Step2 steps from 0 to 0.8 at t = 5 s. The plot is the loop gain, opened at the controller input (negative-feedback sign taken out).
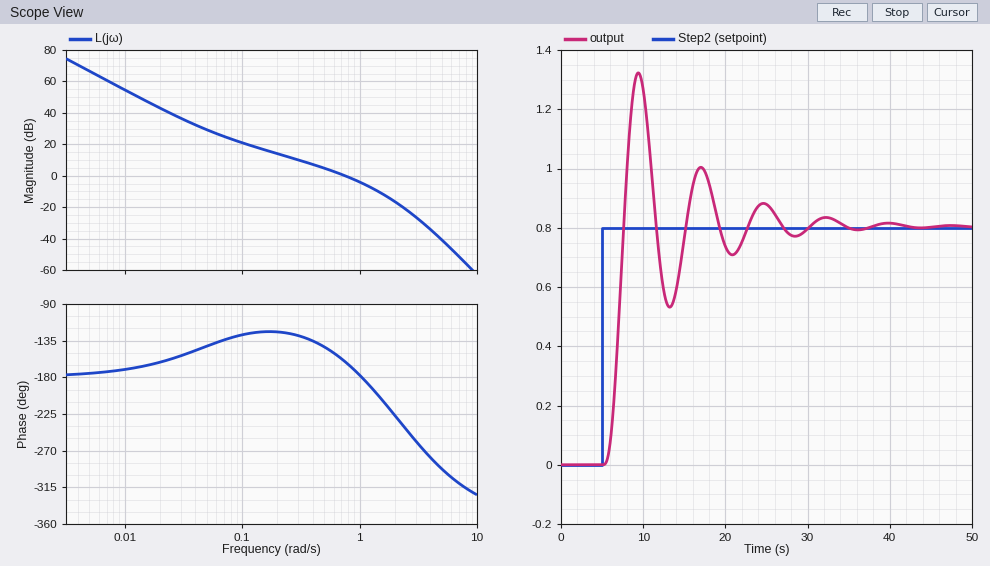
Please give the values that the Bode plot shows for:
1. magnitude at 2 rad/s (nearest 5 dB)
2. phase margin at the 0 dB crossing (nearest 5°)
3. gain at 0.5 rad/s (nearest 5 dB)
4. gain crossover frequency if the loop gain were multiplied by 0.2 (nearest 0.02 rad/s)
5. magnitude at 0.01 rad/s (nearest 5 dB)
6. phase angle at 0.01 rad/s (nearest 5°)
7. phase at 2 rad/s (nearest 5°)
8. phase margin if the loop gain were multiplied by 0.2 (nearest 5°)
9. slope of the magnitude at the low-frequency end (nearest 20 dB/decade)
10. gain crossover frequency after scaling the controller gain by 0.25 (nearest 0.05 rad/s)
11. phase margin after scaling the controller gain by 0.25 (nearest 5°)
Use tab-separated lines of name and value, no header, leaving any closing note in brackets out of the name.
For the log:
magnitude at 2 rad/s	-15 dB
phase margin at the 0 dB crossing	20°
gain at 0.5 rad/s	5 dB
gain crossover frequency if the loop gain were multiplied by 0.2	0.20 rad/s
magnitude at 0.01 rad/s	55 dB
phase angle at 0.01 rad/s	-170°
phase at 2 rad/s	-225°
phase margin if the loop gain were multiplied by 0.2	55°
slope of the magnitude at the low-frequency end	-40 dB/decade
gain crossover frequency after scaling the controller gain by 0.25	0.25 rad/s
phase margin after scaling the controller gain by 0.25	55°
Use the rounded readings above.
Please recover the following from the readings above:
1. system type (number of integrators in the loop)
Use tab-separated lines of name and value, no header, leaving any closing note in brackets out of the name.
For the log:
system type	2
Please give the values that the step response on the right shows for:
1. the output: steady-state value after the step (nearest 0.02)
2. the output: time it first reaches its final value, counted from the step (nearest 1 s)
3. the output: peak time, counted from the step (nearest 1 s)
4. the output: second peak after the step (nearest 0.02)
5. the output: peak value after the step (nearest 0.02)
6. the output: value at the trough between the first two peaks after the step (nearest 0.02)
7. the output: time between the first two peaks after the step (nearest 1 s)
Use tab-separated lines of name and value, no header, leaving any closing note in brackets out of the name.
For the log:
the output: steady-state value after the step	0.80
the output: time it first reaches its final value, counted from the step	3 s
the output: peak time, counted from the step	4 s
the output: second peak after the step	1.00
the output: peak value after the step	1.32
the output: value at the trough between the first two peaks after the step	0.54
the output: time between the first two peaks after the step	8 s
